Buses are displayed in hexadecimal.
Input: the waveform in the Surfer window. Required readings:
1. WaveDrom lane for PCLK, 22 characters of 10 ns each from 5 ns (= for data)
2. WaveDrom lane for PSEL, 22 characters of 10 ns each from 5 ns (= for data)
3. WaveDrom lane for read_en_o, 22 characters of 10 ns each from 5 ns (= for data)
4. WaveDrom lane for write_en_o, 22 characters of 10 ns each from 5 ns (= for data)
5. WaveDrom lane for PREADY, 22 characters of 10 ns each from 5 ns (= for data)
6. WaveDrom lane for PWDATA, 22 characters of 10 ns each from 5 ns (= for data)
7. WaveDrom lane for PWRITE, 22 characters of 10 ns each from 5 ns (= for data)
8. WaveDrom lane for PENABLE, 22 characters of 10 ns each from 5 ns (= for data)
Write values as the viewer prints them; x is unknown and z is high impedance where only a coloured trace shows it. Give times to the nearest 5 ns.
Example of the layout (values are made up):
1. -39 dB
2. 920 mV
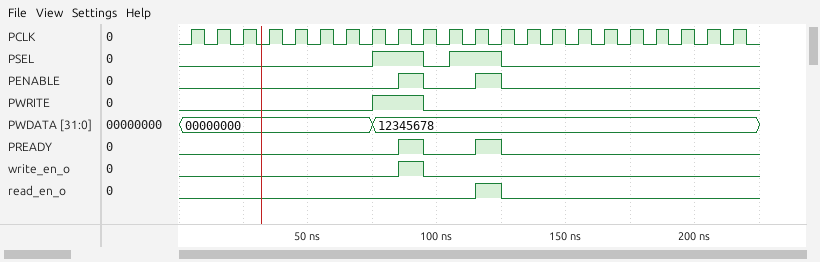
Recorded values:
1. {name: 'PCLK', wave: 'p.....................'}
2. {name: 'PSEL', wave: '0......1.01.0.........'}
3. {name: 'read_en_o', wave: '0..........10.........'}
4. {name: 'write_en_o', wave: '0.......10............'}
5. {name: 'PREADY', wave: '0.......10.10.........'}
6. {name: 'PWDATA', wave: '=......=..............', data: '00000000 12345678'}
7. {name: 'PWRITE', wave: '0......1.0............'}
8. {name: 'PENABLE', wave: '0.......10.10.........'}
